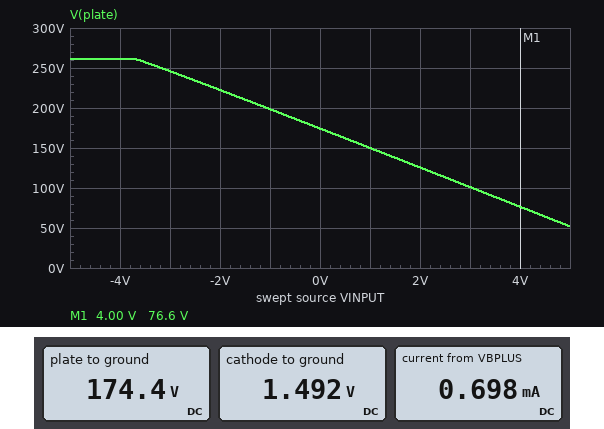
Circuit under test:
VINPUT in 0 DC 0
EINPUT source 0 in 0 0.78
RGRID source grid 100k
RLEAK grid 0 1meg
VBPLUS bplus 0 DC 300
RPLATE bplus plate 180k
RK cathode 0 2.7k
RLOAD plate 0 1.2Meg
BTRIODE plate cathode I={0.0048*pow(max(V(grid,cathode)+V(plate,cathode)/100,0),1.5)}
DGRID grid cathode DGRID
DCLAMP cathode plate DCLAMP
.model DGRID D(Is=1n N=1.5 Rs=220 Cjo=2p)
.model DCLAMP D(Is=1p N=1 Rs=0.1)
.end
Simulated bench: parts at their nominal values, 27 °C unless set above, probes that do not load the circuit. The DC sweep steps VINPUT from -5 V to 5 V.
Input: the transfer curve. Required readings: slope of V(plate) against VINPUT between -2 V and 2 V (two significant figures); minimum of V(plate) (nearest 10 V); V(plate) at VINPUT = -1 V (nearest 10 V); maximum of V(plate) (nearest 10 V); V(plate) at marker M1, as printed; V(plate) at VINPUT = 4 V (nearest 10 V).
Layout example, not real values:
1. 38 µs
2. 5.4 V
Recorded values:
1. -24 V/V
2. 50 V
3. 200 V
4. 260 V
5. 76.6 V
6. 80 V
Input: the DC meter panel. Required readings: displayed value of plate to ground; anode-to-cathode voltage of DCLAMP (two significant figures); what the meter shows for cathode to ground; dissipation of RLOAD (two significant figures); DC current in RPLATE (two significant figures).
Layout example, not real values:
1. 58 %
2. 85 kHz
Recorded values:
1. 174.4 V
2. -170 V
3. 1.492 V
4. 25 mW
5. 700 µA
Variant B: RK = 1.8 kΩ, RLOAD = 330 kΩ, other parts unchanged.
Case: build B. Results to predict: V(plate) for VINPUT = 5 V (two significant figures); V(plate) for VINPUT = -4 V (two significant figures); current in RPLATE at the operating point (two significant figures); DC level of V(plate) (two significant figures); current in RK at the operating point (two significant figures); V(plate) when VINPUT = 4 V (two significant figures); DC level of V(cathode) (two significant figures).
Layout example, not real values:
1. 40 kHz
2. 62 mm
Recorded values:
1. 16 V
2. 190 V
3. 960 µA
4. 130 V
5. 570 µA
6. 26 V
7. 1.0 V
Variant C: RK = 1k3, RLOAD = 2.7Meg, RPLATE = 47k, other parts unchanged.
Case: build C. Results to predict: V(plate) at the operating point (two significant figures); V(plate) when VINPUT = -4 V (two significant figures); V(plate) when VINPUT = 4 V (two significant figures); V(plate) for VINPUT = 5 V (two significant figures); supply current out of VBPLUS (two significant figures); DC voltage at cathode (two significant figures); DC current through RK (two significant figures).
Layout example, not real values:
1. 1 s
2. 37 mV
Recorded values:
1. 230 V
2. 290 V
3. 160 V
4. 150 V
5. 1.5 mA
6. 1.8 V
7. 1.4 mA
